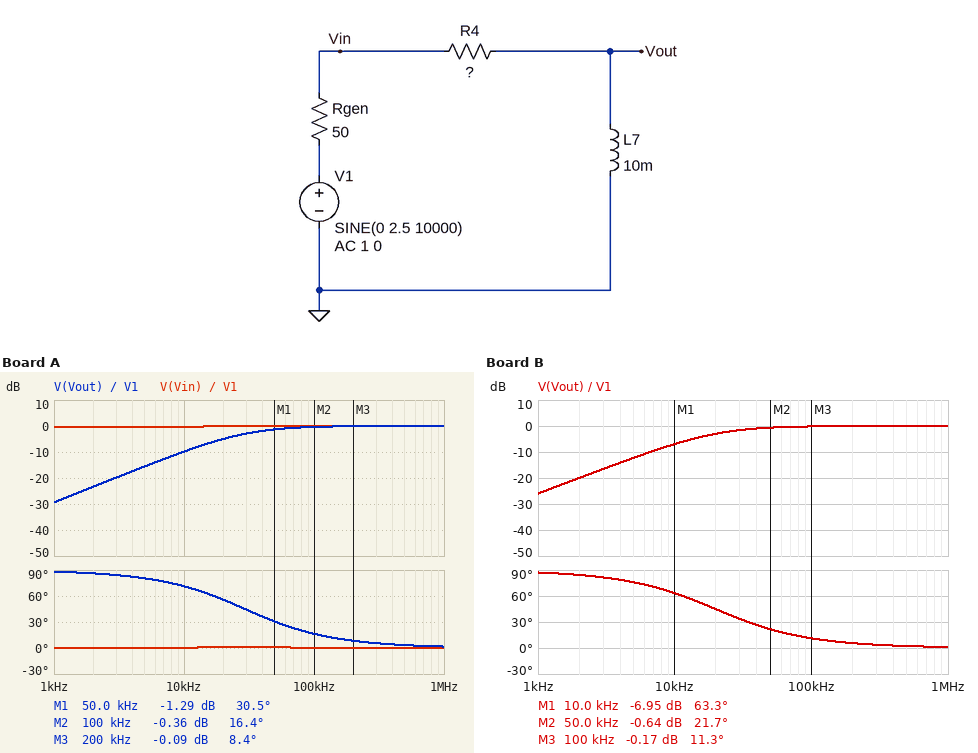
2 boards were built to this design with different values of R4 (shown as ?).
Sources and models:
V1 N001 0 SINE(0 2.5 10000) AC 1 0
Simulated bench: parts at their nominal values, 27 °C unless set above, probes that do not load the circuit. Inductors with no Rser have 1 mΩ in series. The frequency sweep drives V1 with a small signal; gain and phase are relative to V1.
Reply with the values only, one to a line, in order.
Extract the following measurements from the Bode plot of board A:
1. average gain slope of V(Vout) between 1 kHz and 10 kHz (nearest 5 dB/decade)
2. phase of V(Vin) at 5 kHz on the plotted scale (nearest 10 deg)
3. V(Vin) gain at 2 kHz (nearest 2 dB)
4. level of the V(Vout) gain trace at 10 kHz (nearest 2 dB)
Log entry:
20 dB/decade
0 deg
0 dB
-10 dB
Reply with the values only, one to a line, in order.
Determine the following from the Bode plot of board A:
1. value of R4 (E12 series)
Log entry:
1.8 kΩ
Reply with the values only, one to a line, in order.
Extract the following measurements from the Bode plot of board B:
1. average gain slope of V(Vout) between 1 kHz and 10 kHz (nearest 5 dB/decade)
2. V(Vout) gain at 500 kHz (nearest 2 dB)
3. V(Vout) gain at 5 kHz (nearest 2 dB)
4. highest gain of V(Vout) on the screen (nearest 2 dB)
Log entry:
20 dB/decade
0 dB
-12 dB
0 dB
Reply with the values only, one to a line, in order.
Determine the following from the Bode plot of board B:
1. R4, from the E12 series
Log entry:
1.2 kΩ
